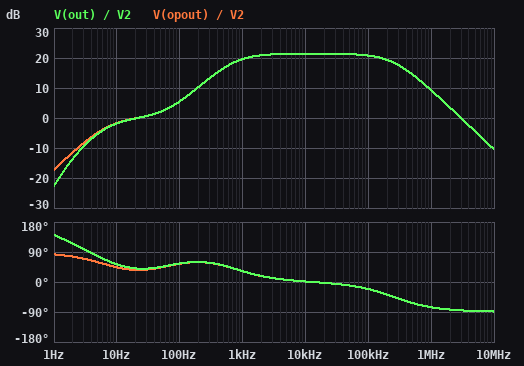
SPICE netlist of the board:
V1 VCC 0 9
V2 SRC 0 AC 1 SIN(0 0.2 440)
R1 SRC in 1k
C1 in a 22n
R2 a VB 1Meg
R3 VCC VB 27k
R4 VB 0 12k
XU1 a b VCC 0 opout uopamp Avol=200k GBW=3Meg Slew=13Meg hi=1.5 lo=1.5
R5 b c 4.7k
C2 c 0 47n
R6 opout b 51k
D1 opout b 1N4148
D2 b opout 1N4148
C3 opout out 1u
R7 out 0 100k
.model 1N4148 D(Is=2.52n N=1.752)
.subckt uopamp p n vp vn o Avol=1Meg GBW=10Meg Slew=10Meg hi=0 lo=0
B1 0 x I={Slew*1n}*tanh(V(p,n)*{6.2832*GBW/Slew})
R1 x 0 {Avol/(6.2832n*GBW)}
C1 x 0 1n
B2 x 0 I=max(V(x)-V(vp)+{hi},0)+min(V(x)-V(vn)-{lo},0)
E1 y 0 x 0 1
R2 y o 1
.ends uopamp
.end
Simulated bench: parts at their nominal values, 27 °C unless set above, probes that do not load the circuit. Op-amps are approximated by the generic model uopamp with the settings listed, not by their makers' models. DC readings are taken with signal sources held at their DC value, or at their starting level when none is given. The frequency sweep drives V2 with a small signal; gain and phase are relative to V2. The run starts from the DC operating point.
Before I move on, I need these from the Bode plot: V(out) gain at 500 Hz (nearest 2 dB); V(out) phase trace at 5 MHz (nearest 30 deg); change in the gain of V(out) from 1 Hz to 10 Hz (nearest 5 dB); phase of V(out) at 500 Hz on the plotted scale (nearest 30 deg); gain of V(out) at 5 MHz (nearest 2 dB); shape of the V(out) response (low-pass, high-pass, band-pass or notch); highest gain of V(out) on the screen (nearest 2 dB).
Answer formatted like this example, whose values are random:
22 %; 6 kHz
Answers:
16 dB; -90 deg; 20 dB; 60 deg; -4 dB; band-pass; 22 dB
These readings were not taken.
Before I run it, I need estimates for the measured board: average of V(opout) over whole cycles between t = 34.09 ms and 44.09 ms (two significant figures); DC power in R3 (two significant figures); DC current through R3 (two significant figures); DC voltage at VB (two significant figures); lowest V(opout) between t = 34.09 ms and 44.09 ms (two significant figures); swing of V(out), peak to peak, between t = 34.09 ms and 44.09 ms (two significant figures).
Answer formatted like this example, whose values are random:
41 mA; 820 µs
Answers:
2.8 V; 1.4 mW; 230 µA; 2.8 V; 2.2 V; 1.1 V
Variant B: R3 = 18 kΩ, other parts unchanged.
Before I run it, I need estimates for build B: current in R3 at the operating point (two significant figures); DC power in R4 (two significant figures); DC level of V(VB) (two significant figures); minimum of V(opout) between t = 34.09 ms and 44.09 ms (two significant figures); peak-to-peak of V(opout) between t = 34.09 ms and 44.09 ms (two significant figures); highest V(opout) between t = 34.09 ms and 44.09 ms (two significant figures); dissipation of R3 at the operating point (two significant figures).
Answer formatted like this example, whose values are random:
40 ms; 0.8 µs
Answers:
300 µA; 1.1 mW; 3.6 V; 3.0 V; 1.1 V; 4.2 V; 1.6 mW
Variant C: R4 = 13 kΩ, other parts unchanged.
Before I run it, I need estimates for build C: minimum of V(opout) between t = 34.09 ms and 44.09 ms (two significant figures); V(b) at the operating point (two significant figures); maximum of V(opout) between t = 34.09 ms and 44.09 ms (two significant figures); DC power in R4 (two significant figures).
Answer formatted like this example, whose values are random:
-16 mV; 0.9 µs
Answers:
2.4 V; 2.9 V; 3.5 V; 660 µW
